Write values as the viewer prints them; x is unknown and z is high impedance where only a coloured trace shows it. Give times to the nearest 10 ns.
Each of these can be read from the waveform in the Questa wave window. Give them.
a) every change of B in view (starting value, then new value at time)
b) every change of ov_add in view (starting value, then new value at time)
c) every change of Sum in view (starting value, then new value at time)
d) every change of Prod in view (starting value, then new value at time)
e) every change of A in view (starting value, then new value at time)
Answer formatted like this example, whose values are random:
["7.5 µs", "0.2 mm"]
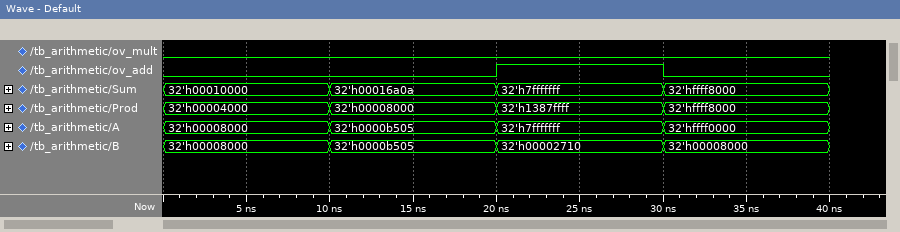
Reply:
["32'h00008000, 32'h0000b505 at 10 ns, 32'h00002710 at 20 ns, 32'h00008000 at 30 ns", "0, 1 at 20 ns, 0 at 30 ns", "32'h00010000, 32'h00016a0a at 10 ns, 32'h7fffffff at 20 ns, 32'hffff8000 at 30 ns", "32'h00004000, 32'h00008000 at 10 ns, 32'h1387ffff at 20 ns, 32'hffff8000 at 30 ns", "32'h00008000, 32'h0000b505 at 10 ns, 32'h7fffffff at 20 ns, 32'hffff0000 at 30 ns"]
